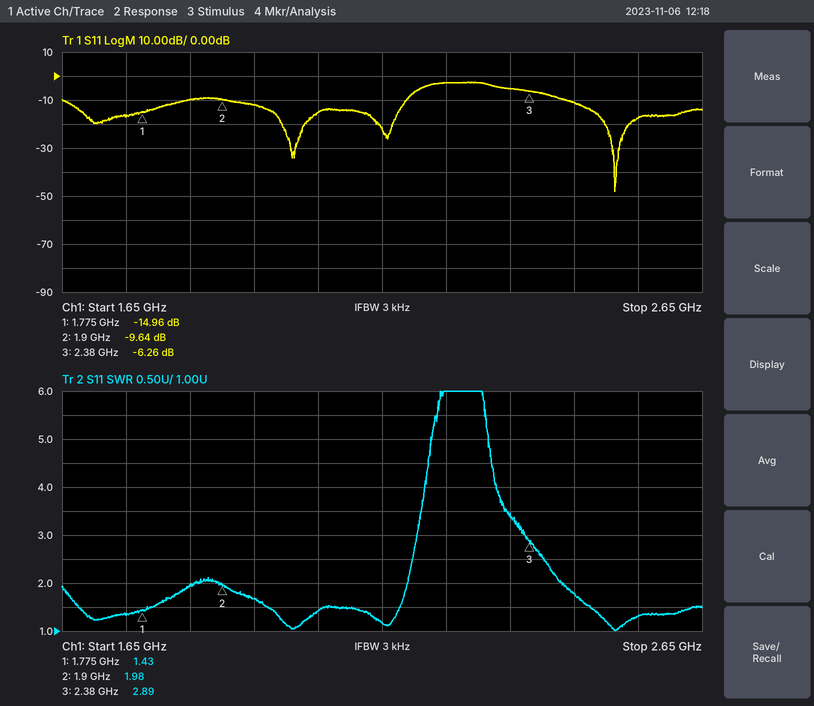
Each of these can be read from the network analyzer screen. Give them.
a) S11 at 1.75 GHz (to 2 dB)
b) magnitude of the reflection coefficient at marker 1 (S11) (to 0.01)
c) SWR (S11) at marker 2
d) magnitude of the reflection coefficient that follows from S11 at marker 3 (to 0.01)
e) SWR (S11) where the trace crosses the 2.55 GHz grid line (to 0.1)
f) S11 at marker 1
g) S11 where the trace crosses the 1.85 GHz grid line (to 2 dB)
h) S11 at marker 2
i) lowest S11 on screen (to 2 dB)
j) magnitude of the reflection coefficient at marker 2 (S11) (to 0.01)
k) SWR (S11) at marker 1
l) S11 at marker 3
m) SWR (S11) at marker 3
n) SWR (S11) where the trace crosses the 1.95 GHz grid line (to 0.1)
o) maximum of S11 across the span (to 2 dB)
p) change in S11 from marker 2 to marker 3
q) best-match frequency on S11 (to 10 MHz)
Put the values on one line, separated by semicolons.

-16 dB; 0.18; 1.98; 0.49; 1.3; -14.96 dB; -10 dB; -9.64 dB; -48 dB; 0.33; 1.43; -6.26 dB; 2.89; 1.7; -2 dB; 3.38 dB; 2.51 GHz
